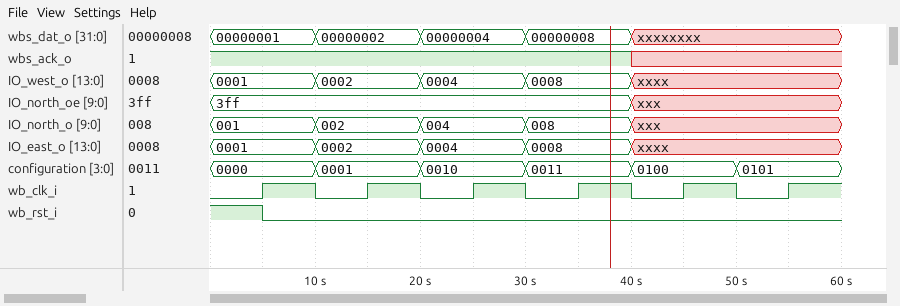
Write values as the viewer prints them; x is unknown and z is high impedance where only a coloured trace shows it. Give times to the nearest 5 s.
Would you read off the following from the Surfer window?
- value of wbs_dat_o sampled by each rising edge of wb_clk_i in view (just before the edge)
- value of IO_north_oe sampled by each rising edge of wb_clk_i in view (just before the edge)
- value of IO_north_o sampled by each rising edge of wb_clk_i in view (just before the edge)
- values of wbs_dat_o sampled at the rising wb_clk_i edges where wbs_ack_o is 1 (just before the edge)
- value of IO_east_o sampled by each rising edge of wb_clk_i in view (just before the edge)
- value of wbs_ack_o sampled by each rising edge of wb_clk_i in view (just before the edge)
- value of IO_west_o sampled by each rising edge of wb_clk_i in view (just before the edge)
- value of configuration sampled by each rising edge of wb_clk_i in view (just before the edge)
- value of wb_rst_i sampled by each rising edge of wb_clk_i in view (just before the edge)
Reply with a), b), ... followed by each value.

a) 00000001, 00000002, 00000004, 00000008, xxxxxxxx, xxxxxxxx
b) 3ff, 3ff, 3ff, 3ff, xxx, xxx
c) 001, 002, 004, 008, xxx, xxx
d) 00000001, 00000002, 00000004, 00000008
e) 0001, 0002, 0004, 0008, xxxx, xxxx
f) 1 1 1 1 x x
g) 0001, 0002, 0004, 0008, xxxx, xxxx
h) 0000, 0001, 0010, 0011, 0100, 0101
i) 1 0 0 0 0 0
